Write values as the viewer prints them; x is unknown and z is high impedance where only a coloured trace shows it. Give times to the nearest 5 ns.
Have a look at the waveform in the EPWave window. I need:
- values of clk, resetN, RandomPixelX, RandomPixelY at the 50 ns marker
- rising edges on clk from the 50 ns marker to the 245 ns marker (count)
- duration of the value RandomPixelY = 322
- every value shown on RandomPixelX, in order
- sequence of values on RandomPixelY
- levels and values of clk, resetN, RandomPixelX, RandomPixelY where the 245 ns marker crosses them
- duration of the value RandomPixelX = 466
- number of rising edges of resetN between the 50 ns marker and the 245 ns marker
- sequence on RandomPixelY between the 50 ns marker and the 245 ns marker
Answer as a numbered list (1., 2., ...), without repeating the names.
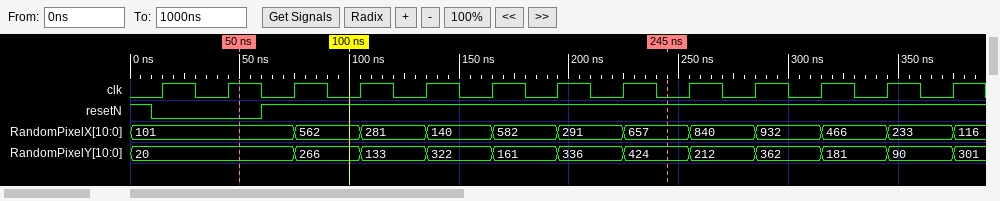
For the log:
1. clk=1, resetN=0, RandomPixelX=101, RandomPixelY=20
2. 6
3. 30 ns
4. 101, 562, 281, 140, 582, 291, 657, 840, 932, 466, 233, 116
5. 20, 266, 133, 322, 161, 336, 424, 212, 362, 181, 90, 301
6. clk=0, resetN=1, RandomPixelX=657, RandomPixelY=424
7. 30 ns
8. 1
9. 20, 266, 133, 322, 161, 336, 424
